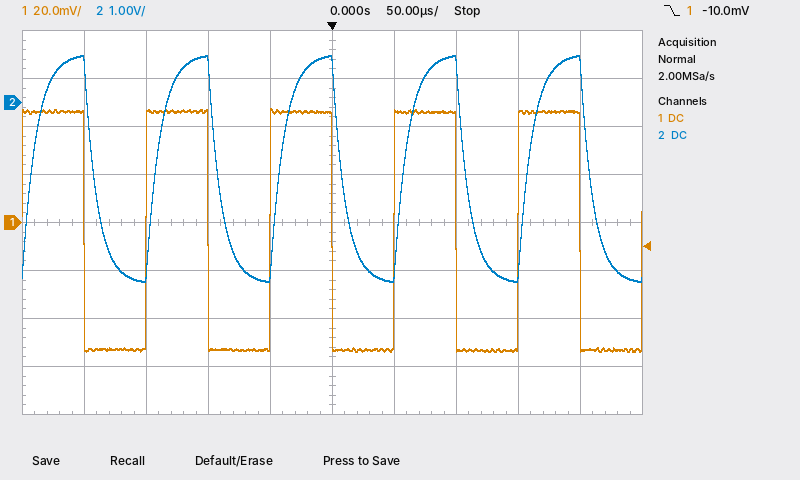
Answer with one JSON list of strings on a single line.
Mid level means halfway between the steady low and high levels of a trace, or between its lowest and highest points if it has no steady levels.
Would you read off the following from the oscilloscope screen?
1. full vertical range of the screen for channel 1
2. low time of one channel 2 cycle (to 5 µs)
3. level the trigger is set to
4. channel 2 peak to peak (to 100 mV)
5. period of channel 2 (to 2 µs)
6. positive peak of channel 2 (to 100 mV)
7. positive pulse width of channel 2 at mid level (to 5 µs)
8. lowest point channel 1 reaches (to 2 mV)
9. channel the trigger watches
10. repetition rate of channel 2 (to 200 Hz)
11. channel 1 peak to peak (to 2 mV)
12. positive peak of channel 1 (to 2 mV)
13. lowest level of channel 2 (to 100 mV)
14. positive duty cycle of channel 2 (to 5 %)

["160 mV", "50 µs", "-10.0 mV", "4.7 V", "100 µs", "1.0 V", "50 µs", "-54 mV", "channel 1", "10.0 kHz", "102 mV", "48 mV", "-3.7 V", "50 %"]
